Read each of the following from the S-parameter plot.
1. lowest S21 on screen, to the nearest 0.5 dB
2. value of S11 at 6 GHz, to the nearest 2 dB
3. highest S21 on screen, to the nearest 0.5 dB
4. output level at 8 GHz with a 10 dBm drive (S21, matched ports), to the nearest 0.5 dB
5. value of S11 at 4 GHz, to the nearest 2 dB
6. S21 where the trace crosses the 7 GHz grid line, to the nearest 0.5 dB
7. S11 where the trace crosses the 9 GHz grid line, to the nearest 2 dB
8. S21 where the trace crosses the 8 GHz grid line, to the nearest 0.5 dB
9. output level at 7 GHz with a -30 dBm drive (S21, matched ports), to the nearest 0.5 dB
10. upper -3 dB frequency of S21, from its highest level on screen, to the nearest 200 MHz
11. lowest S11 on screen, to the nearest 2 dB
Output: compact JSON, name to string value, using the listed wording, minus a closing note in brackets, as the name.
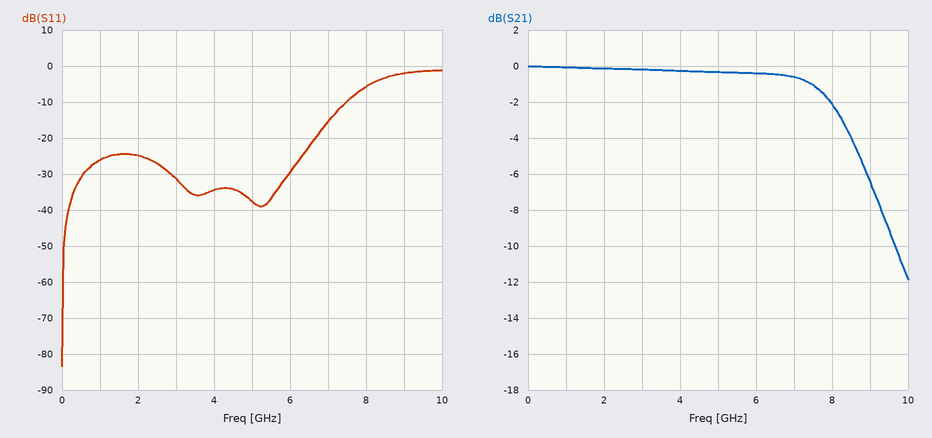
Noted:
{"lowest S21 on screen, to the nearest 0.5 dB": "-12.0 dB", "value of S11 at 6 GHz, to the nearest 2 dB": "-30 dB", "highest S21 on screen, to the nearest 0.5 dB": "0.0 dB", "output level at 8 GHz with a 10 dBm drive (S21, matched ports), to the nearest 0.5 dB": "8.0 dBm", "value of S11 at 4 GHz, to the nearest 2 dB": "-34 dB", "S21 where the trace crosses the 7 GHz grid line, to the nearest 0.5 dB": "-0.5 dB", "S11 where the trace crosses the 9 GHz grid line, to the nearest 2 dB": "-2 dB", "S21 where the trace crosses the 8 GHz grid line, to the nearest 0.5 dB": "-2.0 dB", "output level at 7 GHz with a -30 dBm drive (S21, matched ports), to the nearest 0.5 dB": "-30.5 dBm", "upper -3 dB frequency of S21, from its highest level on screen, to the nearest 200 MHz": "8.2 GHz", "lowest S11 on screen, to the nearest 2 dB": "-84 dB"}
